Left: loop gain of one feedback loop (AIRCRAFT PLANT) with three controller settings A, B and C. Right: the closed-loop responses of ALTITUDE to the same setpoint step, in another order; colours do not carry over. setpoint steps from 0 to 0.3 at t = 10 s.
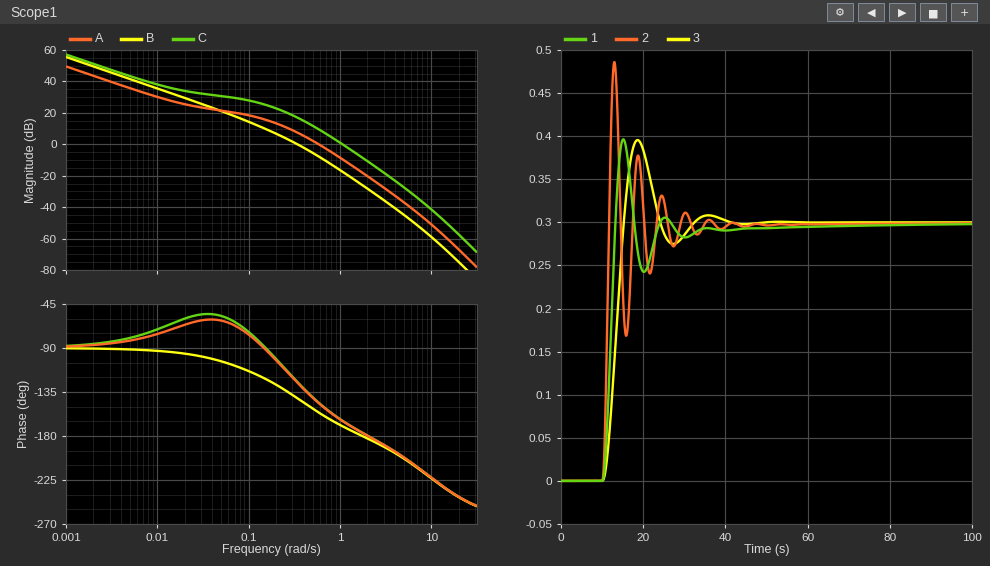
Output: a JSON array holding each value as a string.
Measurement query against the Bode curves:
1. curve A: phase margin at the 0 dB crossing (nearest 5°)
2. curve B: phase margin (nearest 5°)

["35°", "40°"]
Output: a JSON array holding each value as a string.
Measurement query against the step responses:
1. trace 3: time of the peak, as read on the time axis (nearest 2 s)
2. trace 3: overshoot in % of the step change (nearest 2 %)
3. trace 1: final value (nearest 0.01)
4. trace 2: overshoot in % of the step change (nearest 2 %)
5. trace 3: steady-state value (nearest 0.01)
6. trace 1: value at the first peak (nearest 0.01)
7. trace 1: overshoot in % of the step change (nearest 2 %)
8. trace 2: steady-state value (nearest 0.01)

["18 s", "32 %", "0.30", "62 %", "0.30", "0.40", "32 %", "0.30"]
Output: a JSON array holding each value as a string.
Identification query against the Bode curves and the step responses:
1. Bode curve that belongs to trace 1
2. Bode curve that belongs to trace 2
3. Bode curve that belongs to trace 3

["A", "C", "B"]
